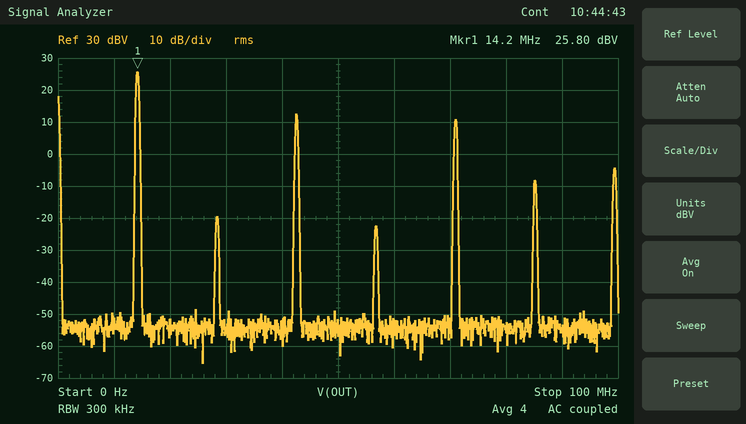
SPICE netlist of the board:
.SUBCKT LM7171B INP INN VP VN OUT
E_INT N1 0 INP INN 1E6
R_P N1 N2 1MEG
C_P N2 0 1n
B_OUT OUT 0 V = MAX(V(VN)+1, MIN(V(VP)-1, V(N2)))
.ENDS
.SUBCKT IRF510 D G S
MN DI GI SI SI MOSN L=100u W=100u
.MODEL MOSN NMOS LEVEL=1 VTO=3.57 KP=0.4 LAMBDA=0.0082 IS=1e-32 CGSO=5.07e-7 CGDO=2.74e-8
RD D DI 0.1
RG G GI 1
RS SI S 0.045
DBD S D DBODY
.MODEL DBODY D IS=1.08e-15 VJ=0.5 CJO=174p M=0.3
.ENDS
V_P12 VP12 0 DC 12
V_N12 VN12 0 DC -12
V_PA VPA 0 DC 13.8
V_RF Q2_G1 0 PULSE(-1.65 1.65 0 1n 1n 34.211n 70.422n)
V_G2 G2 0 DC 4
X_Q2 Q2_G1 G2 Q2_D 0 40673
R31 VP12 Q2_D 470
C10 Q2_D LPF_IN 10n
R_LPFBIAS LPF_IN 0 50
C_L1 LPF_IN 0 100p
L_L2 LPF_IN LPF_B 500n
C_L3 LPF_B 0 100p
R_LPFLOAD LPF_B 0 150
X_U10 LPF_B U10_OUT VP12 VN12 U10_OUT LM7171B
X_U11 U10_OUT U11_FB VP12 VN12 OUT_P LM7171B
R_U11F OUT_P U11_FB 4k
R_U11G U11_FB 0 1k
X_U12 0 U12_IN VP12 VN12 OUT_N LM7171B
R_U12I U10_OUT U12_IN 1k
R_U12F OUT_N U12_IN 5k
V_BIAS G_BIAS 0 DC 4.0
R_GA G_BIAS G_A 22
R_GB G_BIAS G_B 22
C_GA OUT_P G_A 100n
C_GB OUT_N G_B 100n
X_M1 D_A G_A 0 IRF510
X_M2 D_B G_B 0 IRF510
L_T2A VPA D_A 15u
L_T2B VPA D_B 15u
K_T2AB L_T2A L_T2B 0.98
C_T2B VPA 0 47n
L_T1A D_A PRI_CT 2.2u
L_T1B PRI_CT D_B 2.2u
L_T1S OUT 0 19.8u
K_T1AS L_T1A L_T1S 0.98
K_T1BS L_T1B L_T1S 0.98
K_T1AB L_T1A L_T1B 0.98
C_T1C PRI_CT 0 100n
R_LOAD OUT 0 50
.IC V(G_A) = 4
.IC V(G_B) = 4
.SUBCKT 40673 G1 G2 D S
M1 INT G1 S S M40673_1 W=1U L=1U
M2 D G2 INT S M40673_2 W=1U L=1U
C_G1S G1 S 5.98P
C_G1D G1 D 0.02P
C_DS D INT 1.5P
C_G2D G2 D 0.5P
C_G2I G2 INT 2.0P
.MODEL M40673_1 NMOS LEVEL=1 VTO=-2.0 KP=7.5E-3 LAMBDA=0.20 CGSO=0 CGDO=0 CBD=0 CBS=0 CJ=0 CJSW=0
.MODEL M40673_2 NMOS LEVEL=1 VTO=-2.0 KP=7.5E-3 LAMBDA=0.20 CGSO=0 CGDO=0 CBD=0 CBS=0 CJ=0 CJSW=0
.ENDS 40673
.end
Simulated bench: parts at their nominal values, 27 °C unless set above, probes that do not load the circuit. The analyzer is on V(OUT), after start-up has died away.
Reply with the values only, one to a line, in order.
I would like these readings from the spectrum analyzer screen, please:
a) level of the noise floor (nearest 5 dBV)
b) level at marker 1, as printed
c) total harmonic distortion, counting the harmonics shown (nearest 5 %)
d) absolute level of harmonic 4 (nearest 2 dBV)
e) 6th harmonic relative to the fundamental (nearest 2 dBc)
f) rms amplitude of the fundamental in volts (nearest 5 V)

-55 dBV
25.80 dBV
30 %
-22 dBV
-34 dBc
20 V
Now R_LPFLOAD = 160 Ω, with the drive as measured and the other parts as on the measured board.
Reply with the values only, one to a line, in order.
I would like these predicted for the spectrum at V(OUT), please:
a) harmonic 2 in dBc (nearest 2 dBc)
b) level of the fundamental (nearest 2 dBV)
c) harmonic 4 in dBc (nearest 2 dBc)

-48 dBc
26 dBV
-50 dBc
